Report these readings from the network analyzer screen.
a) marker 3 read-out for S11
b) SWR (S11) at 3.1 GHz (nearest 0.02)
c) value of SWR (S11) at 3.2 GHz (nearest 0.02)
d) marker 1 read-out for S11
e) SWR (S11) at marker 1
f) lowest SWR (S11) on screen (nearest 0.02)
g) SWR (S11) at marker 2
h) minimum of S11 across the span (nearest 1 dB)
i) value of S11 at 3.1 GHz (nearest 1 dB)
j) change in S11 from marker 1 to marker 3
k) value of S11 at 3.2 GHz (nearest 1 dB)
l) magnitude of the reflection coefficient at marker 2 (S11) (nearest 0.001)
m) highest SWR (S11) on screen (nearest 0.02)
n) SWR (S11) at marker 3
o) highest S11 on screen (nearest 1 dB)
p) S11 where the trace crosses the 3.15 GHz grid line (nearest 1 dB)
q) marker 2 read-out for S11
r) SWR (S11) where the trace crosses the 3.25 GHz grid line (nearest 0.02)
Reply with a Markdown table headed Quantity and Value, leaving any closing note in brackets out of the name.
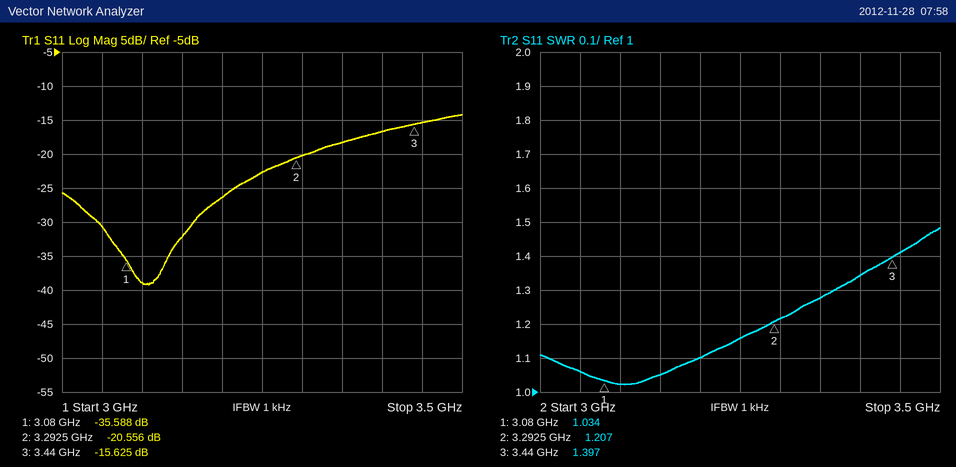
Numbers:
| Quantity | Value |
|---|---|
| marker 3 read-out for S11 | -15.625 dB |
| SWR (S11) at 3.1 GHz | 1.02 |
| value of SWR (S11) at 3.2 GHz | 1.10 |
| marker 1 read-out for S11 | -35.588 dB |
| SWR (S11) at marker 1 | 1.034 |
| lowest SWR (S11) on screen | 1.02 |
| SWR (S11) at marker 2 | 1.207 |
| minimum of S11 across the span | -39 dB |
| value of S11 at 3.1 GHz | -39 dB |
| change in S11 from marker 1 to marker 3 | 19.963 dB |
| value of S11 at 3.2 GHz | -26 dB |
| magnitude of the reflection coefficient at marker 2 (S11) | 0.094 |
| highest SWR (S11) on screen | 1.48 |
| SWR (S11) at marker 3 | 1.397 |
| highest S11 on screen | -14 dB |
| S11 where the trace crosses the 3.15 GHz grid line | -32 dB |
| marker 2 read-out for S11 | -20.556 dB |
| SWR (S11) where the trace crosses the 3.25 GHz grid line | 1.16 |
